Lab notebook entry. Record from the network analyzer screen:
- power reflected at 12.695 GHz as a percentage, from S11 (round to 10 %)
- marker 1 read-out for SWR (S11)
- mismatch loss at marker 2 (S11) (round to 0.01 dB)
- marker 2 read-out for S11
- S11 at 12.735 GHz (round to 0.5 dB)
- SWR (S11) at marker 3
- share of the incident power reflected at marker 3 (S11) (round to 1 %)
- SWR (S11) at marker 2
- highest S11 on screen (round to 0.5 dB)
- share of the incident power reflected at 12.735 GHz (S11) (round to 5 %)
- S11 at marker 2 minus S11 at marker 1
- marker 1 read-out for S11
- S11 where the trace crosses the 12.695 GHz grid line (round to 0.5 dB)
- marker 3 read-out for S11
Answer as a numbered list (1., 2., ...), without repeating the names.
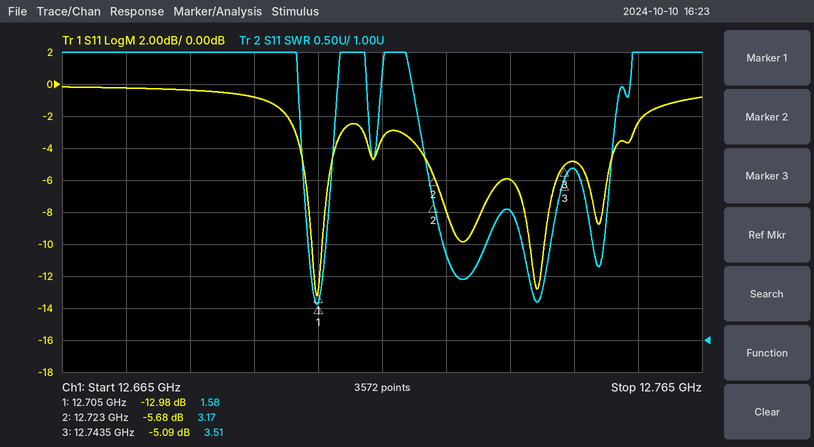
1. 80 %
2. 1.58
3. 1.37 dB
4. -5.68 dB
5. -6.0 dB
6. 3.51
7. 31 %
8. 3.17
9. 0.0 dB
10. 25 %
11. 7.30 dB
12. -12.98 dB
13. -1.0 dB
14. -5.09 dB
